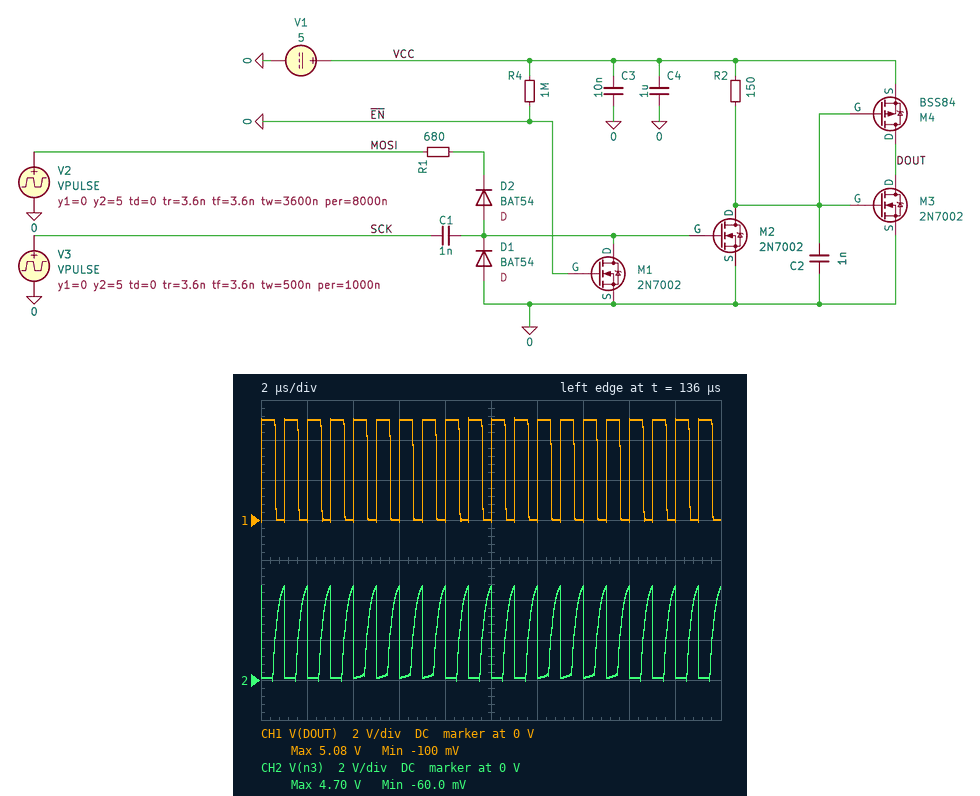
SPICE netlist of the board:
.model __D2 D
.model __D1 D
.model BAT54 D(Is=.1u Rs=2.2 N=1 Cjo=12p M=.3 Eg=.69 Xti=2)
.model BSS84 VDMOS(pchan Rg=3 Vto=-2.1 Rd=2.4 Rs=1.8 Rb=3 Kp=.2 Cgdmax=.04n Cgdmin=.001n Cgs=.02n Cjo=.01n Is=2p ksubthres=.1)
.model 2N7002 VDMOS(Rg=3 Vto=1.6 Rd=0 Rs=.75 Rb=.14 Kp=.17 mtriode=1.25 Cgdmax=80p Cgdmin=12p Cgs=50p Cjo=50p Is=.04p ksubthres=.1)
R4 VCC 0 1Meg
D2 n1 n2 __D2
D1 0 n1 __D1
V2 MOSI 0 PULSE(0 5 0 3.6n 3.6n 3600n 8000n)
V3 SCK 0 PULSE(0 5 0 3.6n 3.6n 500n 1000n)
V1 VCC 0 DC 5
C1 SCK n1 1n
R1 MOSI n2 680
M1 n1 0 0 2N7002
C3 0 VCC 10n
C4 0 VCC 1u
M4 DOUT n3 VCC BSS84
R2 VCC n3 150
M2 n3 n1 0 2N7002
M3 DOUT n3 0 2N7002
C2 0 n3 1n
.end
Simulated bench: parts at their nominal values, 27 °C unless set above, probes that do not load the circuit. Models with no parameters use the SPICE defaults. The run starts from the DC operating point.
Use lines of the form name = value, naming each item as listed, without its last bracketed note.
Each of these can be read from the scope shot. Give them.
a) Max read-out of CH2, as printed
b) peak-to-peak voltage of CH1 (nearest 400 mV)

Max read-out of CH2, as printed = 4.70 V
peak-to-peak voltage of CH1 = 5.2 V
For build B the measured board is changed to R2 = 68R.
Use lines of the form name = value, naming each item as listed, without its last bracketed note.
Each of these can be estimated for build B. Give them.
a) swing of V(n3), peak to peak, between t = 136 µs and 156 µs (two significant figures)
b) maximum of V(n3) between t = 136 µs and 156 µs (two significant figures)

swing of V(n3), peak to peak, between t = 136 µs and 156 µs = 4.9 V
maximum of V(n3) between t = 136 µs and 156 µs = 5.0 V
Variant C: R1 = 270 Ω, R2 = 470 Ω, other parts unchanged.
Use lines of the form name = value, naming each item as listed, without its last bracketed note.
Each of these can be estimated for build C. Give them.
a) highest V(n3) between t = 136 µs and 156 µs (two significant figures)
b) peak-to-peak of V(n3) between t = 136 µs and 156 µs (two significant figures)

highest V(n3) between t = 136 µs and 156 µs = 3.4 V
peak-to-peak of V(n3) between t = 136 µs and 156 µs = 3.6 V
